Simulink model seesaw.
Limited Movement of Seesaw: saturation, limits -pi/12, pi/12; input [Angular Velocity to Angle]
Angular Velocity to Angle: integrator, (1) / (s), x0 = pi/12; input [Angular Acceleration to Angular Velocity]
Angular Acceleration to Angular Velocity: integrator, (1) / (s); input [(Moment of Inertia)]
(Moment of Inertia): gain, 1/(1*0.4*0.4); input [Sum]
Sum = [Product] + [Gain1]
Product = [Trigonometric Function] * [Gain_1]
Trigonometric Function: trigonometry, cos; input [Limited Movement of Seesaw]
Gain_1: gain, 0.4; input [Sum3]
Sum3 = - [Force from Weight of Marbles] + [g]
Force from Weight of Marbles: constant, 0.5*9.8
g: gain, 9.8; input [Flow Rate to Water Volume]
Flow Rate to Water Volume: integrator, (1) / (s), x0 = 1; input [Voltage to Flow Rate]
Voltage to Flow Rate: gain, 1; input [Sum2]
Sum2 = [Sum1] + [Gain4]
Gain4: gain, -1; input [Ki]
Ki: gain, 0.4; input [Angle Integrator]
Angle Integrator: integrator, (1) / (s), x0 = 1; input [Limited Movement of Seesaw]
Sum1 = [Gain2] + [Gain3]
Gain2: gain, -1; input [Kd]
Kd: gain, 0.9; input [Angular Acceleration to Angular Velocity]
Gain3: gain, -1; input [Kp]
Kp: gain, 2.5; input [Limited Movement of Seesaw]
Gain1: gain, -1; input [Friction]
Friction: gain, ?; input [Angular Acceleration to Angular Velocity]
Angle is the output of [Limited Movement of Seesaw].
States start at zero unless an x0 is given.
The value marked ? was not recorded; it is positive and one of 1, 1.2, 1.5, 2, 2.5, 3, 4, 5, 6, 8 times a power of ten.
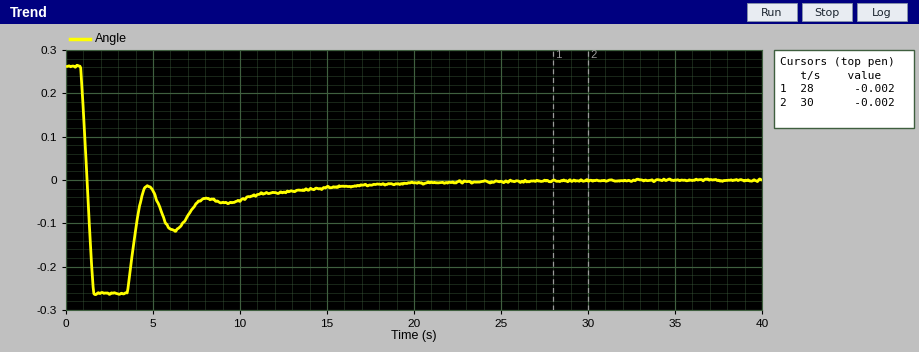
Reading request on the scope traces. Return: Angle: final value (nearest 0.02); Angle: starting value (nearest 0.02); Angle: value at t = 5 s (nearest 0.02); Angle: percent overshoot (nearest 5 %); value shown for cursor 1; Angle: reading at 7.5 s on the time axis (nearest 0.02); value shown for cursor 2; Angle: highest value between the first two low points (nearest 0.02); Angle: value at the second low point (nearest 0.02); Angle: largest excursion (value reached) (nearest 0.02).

0.00
0.26
-0.02
100 %
-0.002
-0.06
-0.002
-0.02
-0.12
-0.26
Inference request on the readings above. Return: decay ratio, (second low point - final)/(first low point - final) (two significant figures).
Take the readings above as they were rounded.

0.46
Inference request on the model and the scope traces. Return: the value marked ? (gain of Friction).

2.5
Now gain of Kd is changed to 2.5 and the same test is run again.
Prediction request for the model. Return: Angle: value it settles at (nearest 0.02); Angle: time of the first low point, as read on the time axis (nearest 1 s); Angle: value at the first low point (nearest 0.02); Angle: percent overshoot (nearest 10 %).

0.00
3 s
-0.18
70 %
